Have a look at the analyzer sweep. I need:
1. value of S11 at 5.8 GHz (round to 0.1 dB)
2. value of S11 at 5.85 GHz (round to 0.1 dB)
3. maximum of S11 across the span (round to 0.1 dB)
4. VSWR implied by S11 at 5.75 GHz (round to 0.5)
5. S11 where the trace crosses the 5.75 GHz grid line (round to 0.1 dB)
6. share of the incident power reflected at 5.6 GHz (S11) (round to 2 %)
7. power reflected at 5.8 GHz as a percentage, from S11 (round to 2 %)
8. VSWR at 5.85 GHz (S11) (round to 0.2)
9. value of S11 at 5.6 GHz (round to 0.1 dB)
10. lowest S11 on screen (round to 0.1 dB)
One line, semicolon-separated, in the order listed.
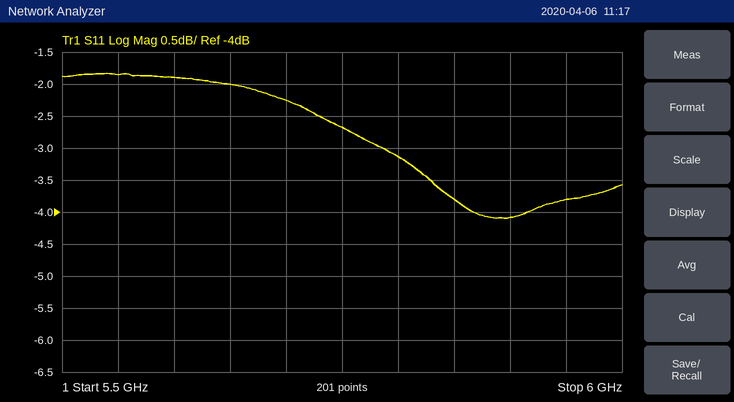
-3.1 dB; -3.8 dB; -1.8 dB; 6.5; -2.7 dB; 64 %; 48 %; 4.6; -1.9 dB; -4.1 dB
